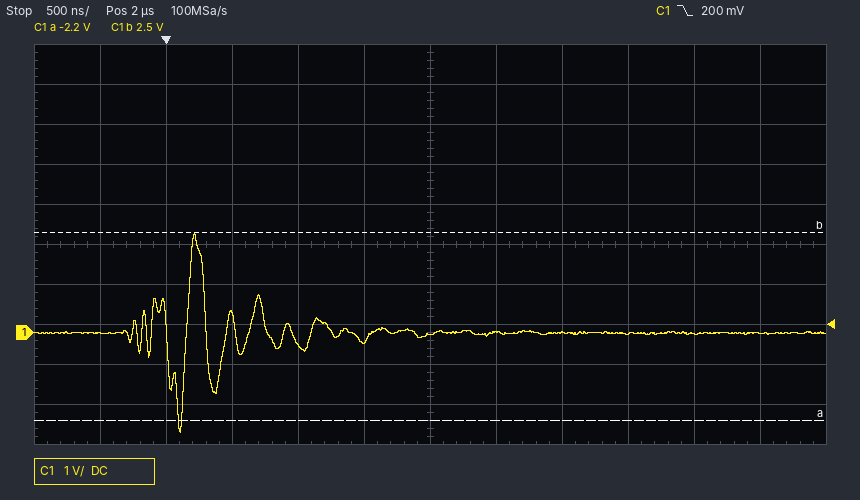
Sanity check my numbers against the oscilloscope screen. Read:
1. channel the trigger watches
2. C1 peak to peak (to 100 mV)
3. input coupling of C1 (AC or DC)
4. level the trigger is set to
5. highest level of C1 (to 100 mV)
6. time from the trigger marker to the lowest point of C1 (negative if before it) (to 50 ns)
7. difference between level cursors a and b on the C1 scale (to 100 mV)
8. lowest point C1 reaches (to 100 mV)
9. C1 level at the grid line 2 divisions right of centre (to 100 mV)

C1
5.0 V
DC
200 mV
2.5 V
+100 ns
4.7 V
-2.5 V
0.0 V
